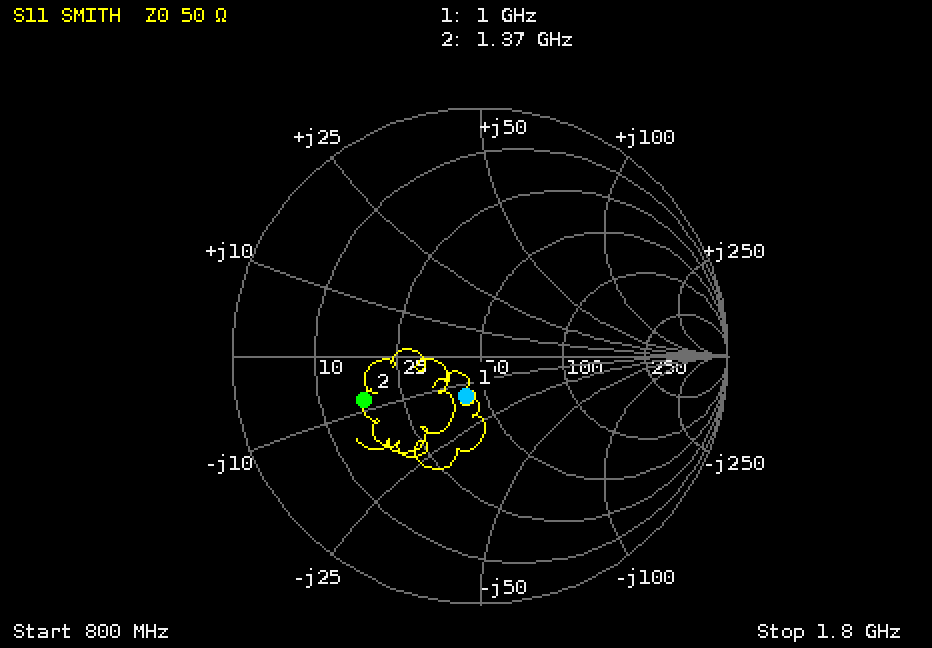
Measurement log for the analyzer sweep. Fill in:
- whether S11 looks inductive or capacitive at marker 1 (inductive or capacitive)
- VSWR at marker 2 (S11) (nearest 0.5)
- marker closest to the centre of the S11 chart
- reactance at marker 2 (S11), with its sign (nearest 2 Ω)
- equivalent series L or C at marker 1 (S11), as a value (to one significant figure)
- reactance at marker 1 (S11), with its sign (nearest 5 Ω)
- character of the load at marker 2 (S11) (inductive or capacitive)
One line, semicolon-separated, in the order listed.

capacitive; 3.0; marker 1; -8 Ω; 10 pF; -15 Ω; capacitive
